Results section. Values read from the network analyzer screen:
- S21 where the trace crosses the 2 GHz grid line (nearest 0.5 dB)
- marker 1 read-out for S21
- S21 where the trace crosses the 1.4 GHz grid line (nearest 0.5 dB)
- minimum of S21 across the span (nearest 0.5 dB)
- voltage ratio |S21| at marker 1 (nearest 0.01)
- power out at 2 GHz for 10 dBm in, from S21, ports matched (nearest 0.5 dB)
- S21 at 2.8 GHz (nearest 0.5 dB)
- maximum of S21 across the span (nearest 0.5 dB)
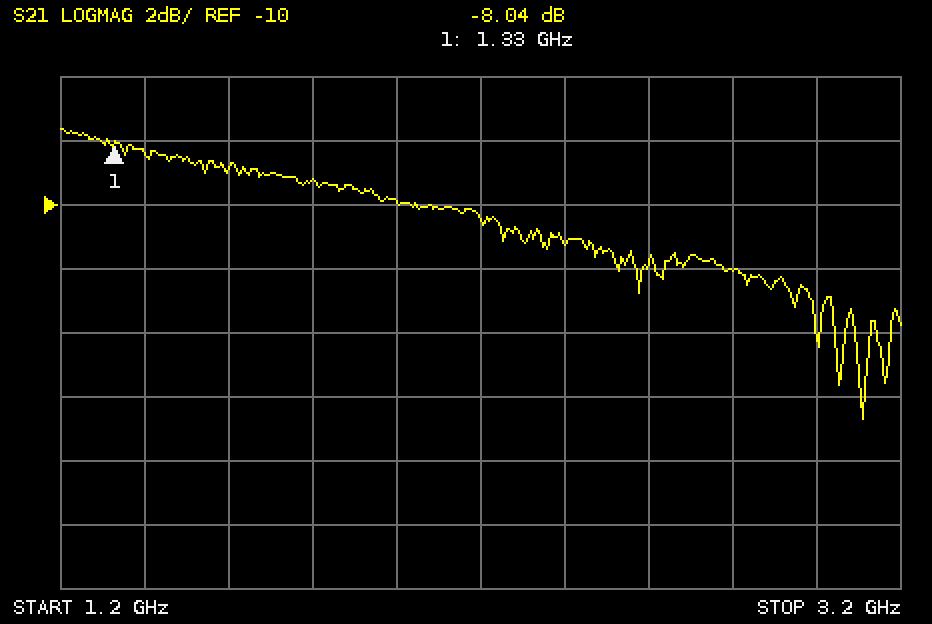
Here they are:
-10.0 dB
-8.04 dB
-8.5 dB
-16.5 dB
0.40
0.0 dBm
-12.0 dB
-7.5 dB
